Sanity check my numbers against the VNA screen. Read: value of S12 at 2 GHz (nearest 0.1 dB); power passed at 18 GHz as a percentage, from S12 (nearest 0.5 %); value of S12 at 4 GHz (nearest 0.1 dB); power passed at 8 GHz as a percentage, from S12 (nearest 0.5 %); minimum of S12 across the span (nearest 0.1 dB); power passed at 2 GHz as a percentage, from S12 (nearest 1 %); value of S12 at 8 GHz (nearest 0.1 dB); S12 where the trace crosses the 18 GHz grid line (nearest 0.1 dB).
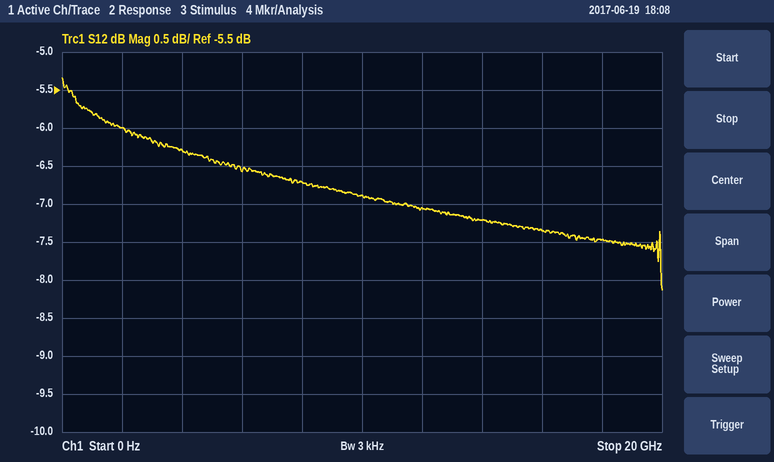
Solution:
-6.0 dB
18.0 %
-6.3 dB
21.5 %
-8.1 dB
25 %
-6.7 dB
-7.5 dB
